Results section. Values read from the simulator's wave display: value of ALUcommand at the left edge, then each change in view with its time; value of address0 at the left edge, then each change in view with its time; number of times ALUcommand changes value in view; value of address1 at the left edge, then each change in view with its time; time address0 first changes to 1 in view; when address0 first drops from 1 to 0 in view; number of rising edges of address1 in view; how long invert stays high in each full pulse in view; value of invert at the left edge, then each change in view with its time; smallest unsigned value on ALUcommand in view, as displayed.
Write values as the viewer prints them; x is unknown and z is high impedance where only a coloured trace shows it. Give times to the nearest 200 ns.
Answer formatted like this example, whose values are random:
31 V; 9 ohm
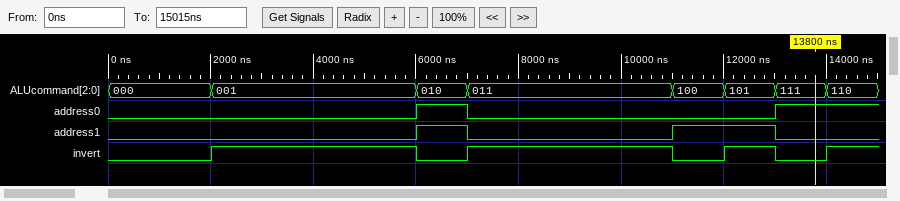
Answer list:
000, 001 at 2000 ns, 010 at 6000 ns, 011 at 7000 ns, 100 at 11000 ns, 101 at 12000 ns, 111 at 13000 ns, 110 at 14000 ns; 0, 1 at 6000 ns, 0 at 7000 ns, 1 at 13000 ns; 7; 0, 1 at 6000 ns, 0 at 7000 ns, 1 at 11000 ns, 0 at 13000 ns; 6000 ns; 7000 ns; 2; 4000 ns, 4000 ns, 1000 ns; 0, 1 at 2000 ns, 0 at 6000 ns, 1 at 7000 ns, 0 at 11000 ns, 1 at 12000 ns, 0 at 13000 ns, 1 at 14000 ns; 000
